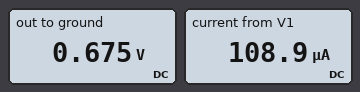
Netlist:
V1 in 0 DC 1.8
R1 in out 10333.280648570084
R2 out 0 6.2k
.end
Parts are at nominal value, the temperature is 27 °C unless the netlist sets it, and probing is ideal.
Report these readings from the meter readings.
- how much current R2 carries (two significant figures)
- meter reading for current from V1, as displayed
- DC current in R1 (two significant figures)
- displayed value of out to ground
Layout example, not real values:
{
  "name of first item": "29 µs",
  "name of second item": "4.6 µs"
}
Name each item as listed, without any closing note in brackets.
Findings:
{
  "how much current R2 carries": "110 µA",
  "meter reading for current from V1, as displayed": "108.9 µA",
  "DC current in R1": "110 µA",
  "displayed value of out to ground": "0.675 V"
}
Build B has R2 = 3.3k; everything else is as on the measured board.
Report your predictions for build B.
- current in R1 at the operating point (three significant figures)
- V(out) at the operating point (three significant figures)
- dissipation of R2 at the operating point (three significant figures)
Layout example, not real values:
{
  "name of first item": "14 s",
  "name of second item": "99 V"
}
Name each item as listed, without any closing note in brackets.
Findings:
{
  "current in R1 at the operating point": "132 µA",
  "V(out) at the operating point": "436 mV",
  "dissipation of R2 at the operating point": "57.5 µW"
}
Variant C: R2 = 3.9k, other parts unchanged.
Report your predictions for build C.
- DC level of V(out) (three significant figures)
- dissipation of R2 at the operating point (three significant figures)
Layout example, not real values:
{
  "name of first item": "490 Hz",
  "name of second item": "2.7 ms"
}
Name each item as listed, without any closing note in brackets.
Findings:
{
  "DC level of V(out)": "493 mV",
  "dissipation of R2 at the operating point": "62.4 µW"
}
